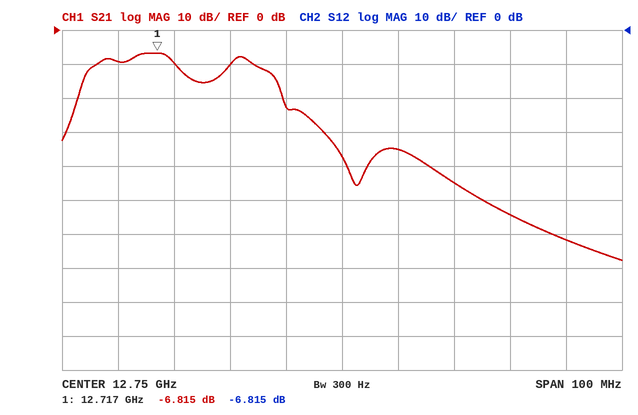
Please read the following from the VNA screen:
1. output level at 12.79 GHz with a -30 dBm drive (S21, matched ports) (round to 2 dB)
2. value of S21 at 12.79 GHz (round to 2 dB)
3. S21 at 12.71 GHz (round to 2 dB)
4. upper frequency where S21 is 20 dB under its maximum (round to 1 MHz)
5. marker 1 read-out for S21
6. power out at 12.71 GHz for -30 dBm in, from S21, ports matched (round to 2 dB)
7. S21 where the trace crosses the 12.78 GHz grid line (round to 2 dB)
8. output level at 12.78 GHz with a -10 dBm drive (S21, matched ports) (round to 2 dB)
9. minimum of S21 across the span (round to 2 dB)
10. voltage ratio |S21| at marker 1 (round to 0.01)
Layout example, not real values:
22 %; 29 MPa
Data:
-92 dBm; -62 dB; -10 dB; 12.745 GHz; -6.815 dB; -40 dBm; -54 dB; -64 dBm; -68 dB; 0.46
